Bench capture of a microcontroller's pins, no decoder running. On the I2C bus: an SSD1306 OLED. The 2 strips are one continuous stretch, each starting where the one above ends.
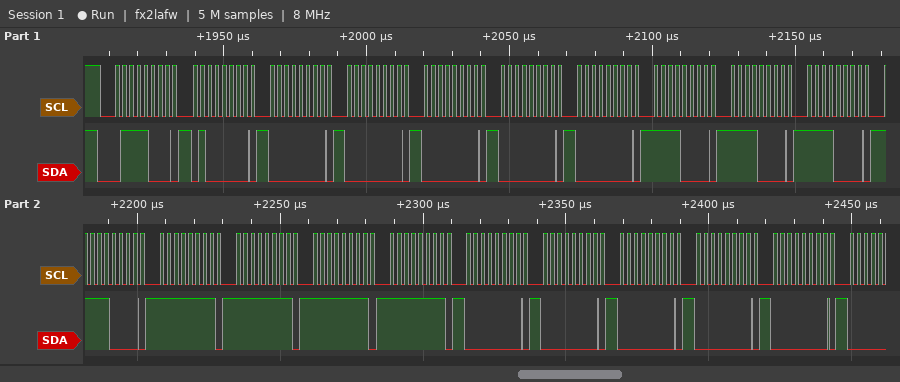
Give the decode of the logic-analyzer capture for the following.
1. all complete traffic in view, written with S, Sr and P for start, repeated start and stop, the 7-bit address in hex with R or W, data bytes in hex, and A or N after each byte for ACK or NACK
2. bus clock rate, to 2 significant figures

S 3CW A 40 A 00 A 00 A 00 A 00 A 00 A F0 A F0 A F0 A F0 A FF A FF A FF A FF A 00 A 00 A 00 A 00 A 00 A
400 kHz
